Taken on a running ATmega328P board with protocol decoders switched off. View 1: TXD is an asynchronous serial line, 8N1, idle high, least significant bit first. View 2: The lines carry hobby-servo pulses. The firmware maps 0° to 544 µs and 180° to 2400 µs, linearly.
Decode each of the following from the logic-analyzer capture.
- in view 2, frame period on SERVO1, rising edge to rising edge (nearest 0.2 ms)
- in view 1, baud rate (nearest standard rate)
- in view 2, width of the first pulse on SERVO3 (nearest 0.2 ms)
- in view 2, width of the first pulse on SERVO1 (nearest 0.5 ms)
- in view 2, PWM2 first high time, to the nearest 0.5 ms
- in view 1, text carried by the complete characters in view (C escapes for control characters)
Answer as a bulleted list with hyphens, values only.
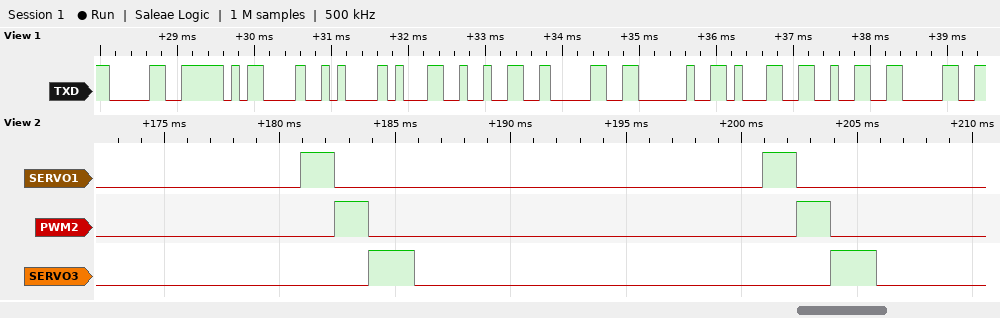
- 20.0 ms
- 9600 baud
- 2.0 ms
- 1.5 ms
- 1.5 ms
- "0\r\n120 120"
